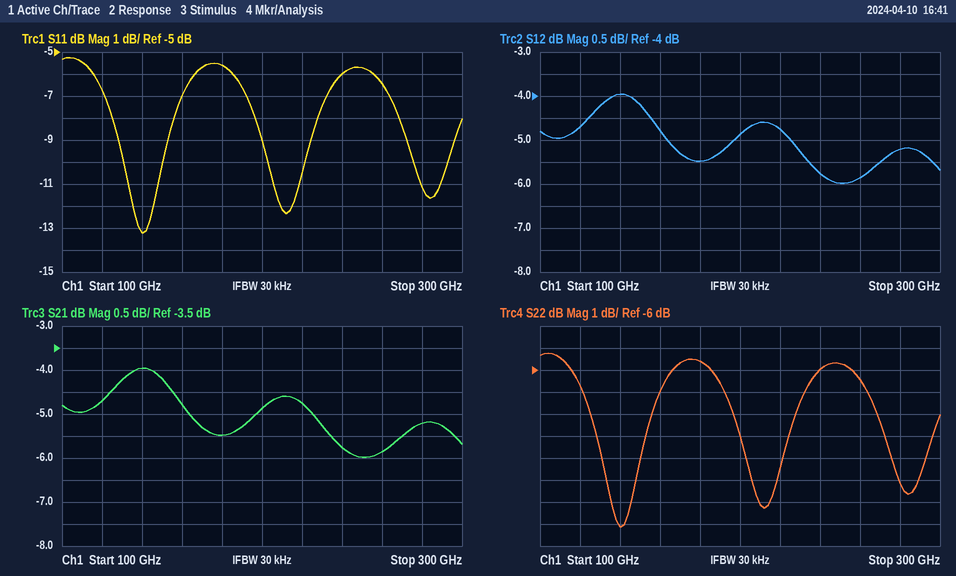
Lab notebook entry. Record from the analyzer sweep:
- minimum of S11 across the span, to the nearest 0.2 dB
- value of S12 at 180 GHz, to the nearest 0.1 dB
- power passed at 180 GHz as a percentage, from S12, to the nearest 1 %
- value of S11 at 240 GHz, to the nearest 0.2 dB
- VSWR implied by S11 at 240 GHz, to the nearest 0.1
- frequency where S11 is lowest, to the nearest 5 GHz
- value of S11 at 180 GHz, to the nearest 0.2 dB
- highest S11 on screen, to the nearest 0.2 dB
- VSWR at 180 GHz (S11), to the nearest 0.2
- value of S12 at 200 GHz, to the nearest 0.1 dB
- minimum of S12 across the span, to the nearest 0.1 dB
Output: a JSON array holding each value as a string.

["-13.2 dB", "-5.5 dB", "28 %", "-6.0 dB", "3.0", "140 GHz", "-5.6 dB", "-5.2 dB", "3.2", "-4.9 dB", "-6.0 dB"]
